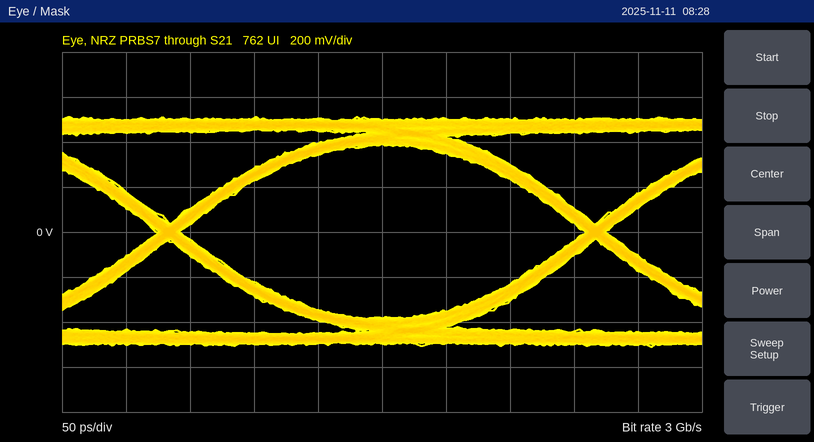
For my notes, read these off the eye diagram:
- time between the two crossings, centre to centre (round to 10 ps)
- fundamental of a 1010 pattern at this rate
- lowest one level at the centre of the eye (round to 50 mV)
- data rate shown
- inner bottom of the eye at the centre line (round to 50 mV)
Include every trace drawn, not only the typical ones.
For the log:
330 ps
1.5 GHz
400 mV
3 Gb/s
-400 mV
